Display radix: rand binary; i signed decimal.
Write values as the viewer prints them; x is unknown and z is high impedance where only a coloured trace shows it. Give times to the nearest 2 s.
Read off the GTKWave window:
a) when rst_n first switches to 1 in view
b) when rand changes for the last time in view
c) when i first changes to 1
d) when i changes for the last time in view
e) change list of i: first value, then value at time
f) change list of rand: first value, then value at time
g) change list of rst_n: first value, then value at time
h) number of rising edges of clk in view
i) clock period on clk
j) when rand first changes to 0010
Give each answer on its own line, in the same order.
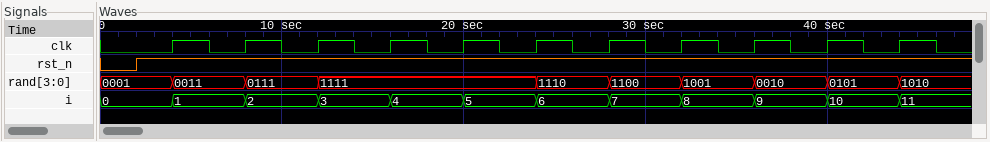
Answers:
2 s
44 s
4 s
44 s
0, 1 at 4 s, 2 at 8 s, 3 at 12 s, 4 at 16 s, 5 at 20 s, 6 at 24 s, 7 at 28 s, 8 at 32 s, 9 at 36 s, 10 at 40 s, 11 at 44 s
0001, 0011 at 4 s, 0111 at 8 s, 1111 at 12 s, 1110 at 24 s, 1100 at 28 s, 1001 at 32 s, 0010 at 36 s, 0101 at 40 s, 1010 at 44 s
0, 1 at 2 s
11
4 s
36 s
